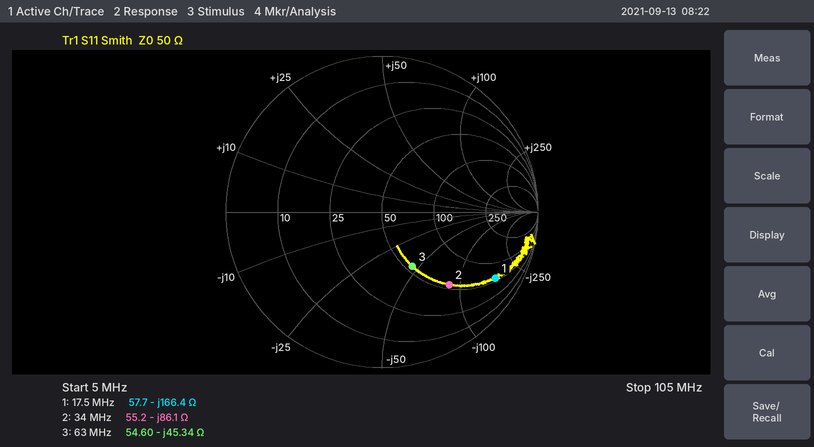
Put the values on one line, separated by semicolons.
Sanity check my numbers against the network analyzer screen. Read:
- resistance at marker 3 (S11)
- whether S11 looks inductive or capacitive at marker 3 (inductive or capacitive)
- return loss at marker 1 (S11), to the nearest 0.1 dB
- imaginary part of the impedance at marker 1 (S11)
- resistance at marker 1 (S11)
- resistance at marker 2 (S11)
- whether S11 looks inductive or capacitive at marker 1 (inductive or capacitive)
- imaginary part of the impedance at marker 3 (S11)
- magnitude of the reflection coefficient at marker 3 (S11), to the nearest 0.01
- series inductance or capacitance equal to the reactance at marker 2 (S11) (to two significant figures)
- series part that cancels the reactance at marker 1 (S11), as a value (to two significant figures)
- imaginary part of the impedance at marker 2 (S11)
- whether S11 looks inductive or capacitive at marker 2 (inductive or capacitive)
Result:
54.60 Ω; capacitive; 1.5 dB; -166.4 Ω; 57.7 Ω; 55.2 Ω; capacitive; -45.34 Ω; 0.40; 54 pF; 1.5 µH; -86.1 Ω; capacitive
